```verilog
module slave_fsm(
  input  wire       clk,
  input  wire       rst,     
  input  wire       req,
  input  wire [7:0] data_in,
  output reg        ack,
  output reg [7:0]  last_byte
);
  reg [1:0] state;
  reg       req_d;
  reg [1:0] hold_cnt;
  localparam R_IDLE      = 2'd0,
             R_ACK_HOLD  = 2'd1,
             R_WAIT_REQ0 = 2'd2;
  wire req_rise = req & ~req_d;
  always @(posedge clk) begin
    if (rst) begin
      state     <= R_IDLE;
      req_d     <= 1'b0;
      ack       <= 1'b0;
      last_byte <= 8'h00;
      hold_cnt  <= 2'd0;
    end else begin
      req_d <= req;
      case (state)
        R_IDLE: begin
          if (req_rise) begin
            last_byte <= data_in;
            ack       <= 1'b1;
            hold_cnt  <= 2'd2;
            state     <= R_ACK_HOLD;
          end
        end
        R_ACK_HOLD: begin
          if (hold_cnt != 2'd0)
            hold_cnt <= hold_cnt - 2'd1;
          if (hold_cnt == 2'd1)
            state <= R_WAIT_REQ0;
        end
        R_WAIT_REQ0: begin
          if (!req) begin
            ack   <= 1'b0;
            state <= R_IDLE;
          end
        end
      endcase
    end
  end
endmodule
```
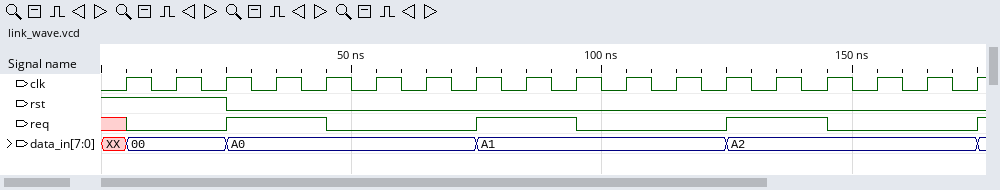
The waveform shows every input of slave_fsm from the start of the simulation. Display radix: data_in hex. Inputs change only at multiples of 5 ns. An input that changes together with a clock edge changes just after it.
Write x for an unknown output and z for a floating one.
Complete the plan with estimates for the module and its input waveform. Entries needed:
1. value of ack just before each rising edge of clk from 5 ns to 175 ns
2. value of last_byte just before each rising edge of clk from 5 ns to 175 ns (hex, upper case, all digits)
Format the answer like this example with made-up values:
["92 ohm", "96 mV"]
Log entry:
["x 0 0 0 1 1 1 0 0 1 1 1 0 0 1 1 1 0", "x, 00, 00, 00, A0, A0, A0, A0, A0, A1, A1, A1, A1, A1, A2, A2, A2, A2"]
